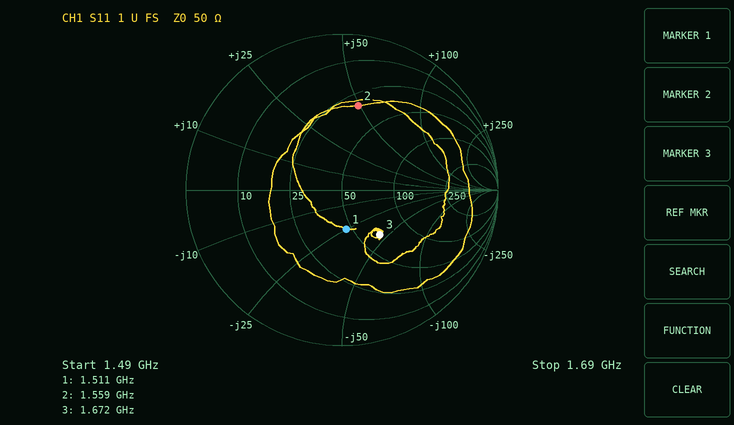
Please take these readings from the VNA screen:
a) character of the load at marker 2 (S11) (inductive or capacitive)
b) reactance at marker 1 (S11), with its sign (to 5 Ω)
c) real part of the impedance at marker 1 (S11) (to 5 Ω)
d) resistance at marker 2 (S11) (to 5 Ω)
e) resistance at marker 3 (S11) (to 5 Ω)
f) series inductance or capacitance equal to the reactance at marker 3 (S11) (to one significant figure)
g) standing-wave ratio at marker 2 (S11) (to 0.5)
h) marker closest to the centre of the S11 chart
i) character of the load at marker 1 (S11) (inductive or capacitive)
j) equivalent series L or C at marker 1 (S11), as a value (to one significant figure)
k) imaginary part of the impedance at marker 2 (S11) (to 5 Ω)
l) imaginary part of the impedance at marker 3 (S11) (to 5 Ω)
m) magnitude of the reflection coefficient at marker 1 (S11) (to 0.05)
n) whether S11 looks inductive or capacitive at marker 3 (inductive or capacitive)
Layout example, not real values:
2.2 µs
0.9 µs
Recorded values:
inductive
-25 Ω
45 Ω
30 Ω
65 Ω
2 pF
3.5
marker 1
capacitive
4 pF
+50 Ω
-45 Ω
0.25
capacitive
